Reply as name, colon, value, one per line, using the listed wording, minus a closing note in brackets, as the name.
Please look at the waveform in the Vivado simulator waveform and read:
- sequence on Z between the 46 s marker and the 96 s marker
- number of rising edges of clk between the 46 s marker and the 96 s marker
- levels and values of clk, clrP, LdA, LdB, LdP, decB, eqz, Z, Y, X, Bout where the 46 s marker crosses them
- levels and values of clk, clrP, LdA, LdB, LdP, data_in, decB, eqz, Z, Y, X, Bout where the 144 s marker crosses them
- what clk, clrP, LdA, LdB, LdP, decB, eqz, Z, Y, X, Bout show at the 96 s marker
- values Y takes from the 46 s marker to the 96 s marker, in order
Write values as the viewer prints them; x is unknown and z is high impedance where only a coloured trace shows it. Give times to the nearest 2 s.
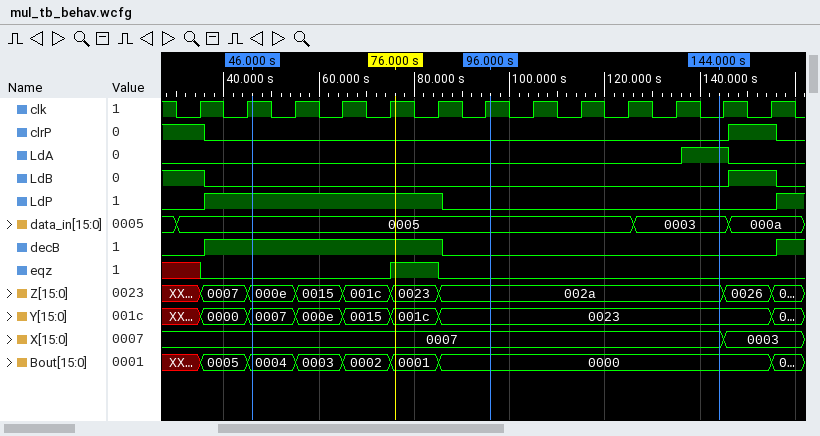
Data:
sequence on Z between the 46 s marker and the 96 s marker: 000e, 0015, 001c, 0023, 002a
number of rising edges of clk between the 46 s marker and the 96 s marker: 5
levels and values of clk, clrP, LdA, LdB, LdP, decB, eqz, Z, Y, X, Bout where the 46 s marker crosses them: clk=1, clrP=0, LdA=0, LdB=0, LdP=1, decB=1, eqz=0, Z=000e, Y=0007, X=0007, Bout=0004
levels and values of clk, clrP, LdA, LdB, LdP, data_in, decB, eqz, Z, Y, X, Bout where the 144 s marker crosses them: clk=0, clrP=0, LdA=1, LdB=0, LdP=0, data_in=0003, decB=0, eqz=0, Z=002a, Y=0023, X=0007, Bout=0000
what clk, clrP, LdA, LdB, LdP, decB, eqz, Z, Y, X, Bout show at the 96 s marker: clk=1, clrP=0, LdA=0, LdB=0, LdP=0, decB=0, eqz=0, Z=002a, Y=0023, X=0007, Bout=0000
values Y takes from the 46 s marker to the 96 s marker, in order: 0007, 000e, 0015, 001c, 0023
